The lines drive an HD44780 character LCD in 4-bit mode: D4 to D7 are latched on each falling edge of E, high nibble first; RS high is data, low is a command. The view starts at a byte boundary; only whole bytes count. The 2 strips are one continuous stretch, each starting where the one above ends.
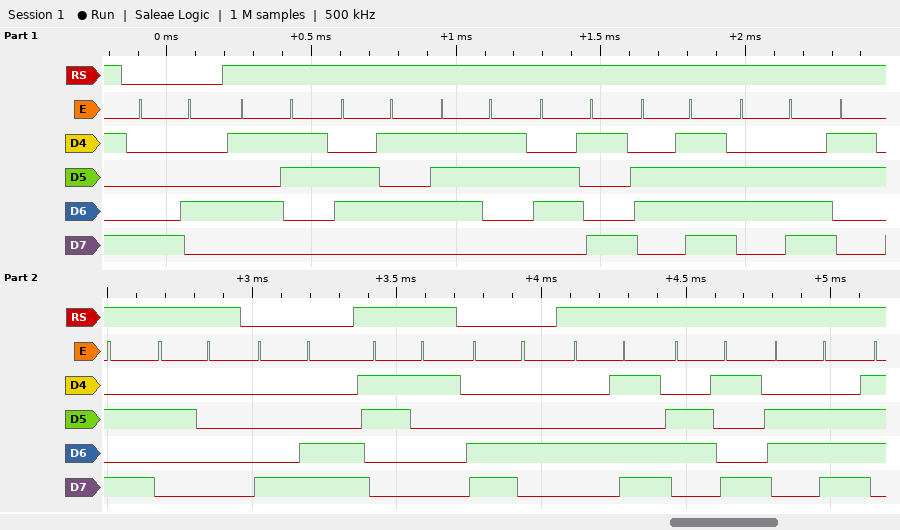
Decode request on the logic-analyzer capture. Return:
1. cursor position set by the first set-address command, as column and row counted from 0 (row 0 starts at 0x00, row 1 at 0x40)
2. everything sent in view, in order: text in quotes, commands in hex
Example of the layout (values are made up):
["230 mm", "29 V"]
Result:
["column 4, row 0", "0x84 \"Sesion: \" 0x8C \"1\" 0xC4 \"Min\""]
